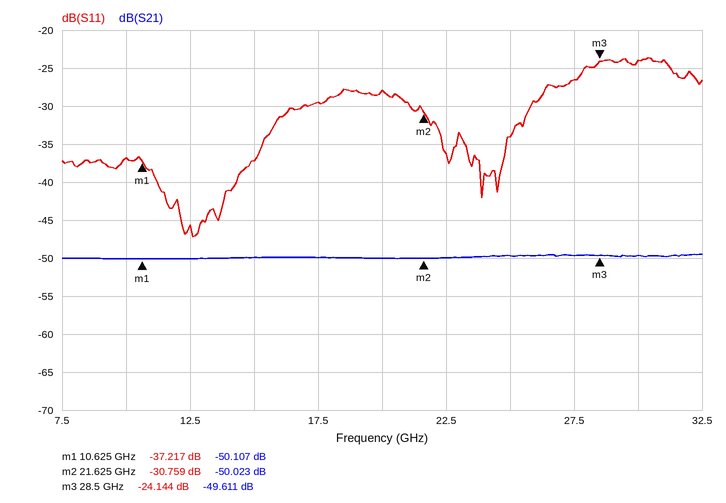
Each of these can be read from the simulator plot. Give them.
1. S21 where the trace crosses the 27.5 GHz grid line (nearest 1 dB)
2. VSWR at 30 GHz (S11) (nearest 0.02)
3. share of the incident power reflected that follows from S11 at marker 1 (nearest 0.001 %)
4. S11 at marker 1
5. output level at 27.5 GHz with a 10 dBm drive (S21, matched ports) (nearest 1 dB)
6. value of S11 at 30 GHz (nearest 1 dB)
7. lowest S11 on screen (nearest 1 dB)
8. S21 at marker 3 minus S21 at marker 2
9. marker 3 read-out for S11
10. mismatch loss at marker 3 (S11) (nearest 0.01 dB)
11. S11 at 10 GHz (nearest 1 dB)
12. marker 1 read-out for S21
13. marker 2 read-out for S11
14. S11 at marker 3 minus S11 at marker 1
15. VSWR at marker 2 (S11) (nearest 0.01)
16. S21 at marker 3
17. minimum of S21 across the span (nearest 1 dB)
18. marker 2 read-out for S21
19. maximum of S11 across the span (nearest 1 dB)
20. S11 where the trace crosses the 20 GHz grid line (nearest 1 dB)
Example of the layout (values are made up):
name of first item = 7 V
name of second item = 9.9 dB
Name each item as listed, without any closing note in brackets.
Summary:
S21 where the trace crosses the 27.5 GHz grid line = -50 dB
VSWR at 30 GHz (S11) = 1.14
share of the incident power reflected that follows from S11 at marker 1 = 0.019 %
S11 at marker 1 = -37.217 dB
output level at 27.5 GHz with a 10 dBm drive (S21, matched ports) = -40 dBm
value of S11 at 30 GHz = -24 dB
lowest S11 on screen = -47 dB
S21 at marker 3 minus S21 at marker 2 = 0.412 dB
marker 3 read-out for S11 = -24.144 dB
mismatch loss at marker 3 (S11) = 0.02 dB
S11 at 10 GHz = -37 dB
marker 1 read-out for S21 = -50.107 dB
marker 2 read-out for S11 = -30.759 dB
S11 at marker 3 minus S11 at marker 1 = 13.073 dB
VSWR at marker 2 (S11) = 1.06
S21 at marker 3 = -49.611 dB
minimum of S21 across the span = -50 dB
marker 2 read-out for S21 = -50.023 dB
maximum of S11 across the span = -24 dB
S11 where the trace crosses the 20 GHz grid line = -28 dB
